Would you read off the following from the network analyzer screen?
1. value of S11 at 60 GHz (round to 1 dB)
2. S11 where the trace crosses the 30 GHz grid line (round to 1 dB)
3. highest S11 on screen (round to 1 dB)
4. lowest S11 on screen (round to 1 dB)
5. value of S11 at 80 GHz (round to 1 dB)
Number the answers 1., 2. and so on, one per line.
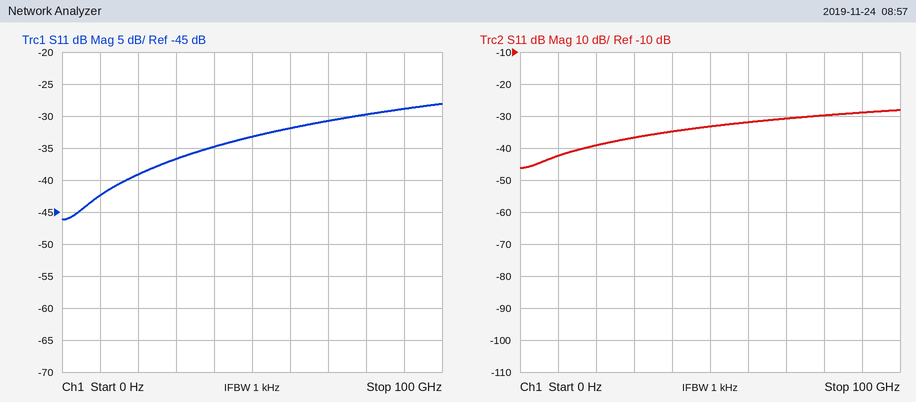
1. -32 dB
2. -37 dB
3. -28 dB
4. -46 dB
5. -30 dB
